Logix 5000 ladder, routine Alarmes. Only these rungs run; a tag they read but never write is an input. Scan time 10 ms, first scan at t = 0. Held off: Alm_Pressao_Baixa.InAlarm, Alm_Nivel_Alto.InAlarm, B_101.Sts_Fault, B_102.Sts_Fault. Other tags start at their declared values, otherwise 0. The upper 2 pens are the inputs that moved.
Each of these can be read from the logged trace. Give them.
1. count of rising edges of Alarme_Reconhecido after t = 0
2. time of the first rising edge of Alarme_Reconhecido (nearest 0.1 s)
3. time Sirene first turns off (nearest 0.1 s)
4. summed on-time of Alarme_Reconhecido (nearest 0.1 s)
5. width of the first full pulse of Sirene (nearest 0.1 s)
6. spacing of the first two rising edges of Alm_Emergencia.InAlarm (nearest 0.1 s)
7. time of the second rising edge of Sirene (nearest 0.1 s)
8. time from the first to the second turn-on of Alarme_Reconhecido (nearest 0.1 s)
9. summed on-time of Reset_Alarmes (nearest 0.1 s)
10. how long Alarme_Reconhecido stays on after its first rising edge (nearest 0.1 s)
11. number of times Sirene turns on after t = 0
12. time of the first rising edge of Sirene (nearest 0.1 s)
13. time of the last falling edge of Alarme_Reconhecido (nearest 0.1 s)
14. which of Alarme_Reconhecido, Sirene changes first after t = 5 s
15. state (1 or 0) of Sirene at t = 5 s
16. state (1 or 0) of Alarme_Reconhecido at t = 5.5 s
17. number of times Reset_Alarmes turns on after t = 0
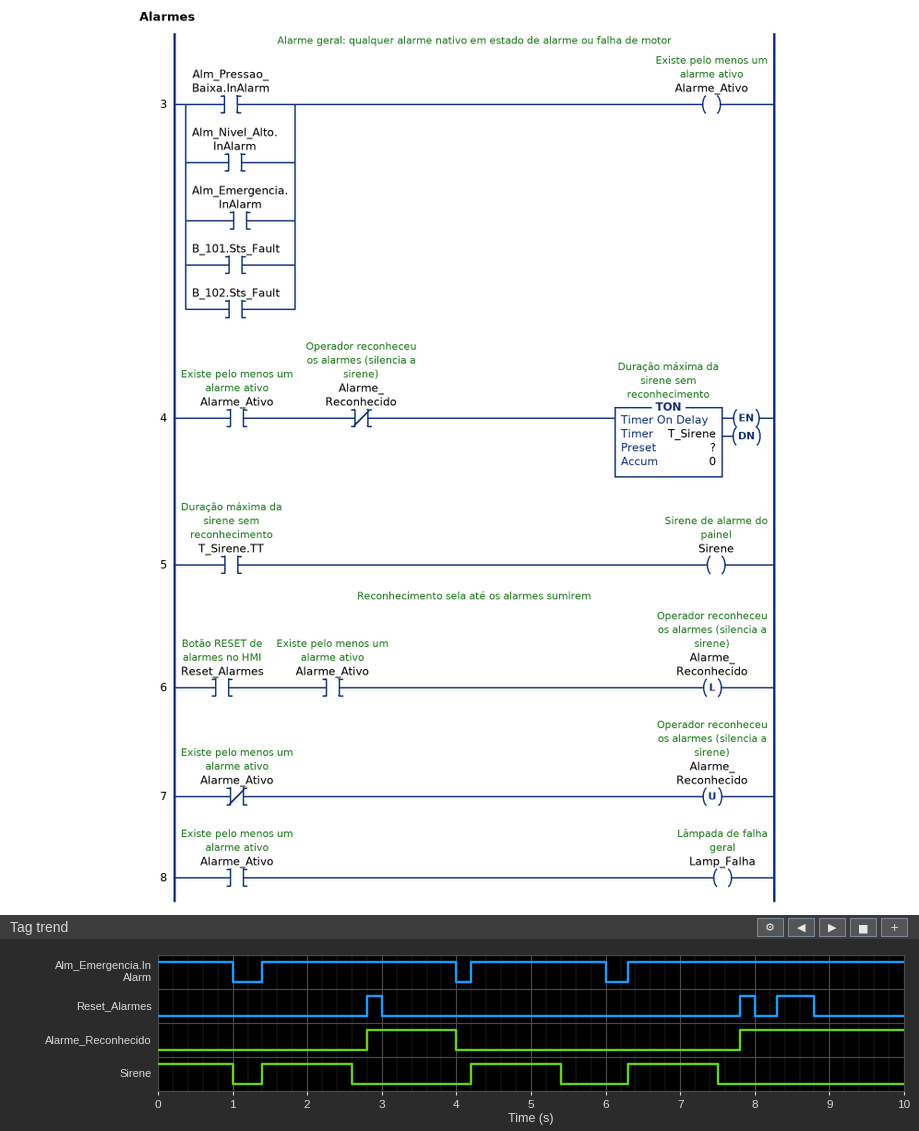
2
2.8 s
1.0 s
3.4 s
1.2 s
2.8 s
4.2 s
5.0 s
0.9 s
1.2 s
3
1.4 s
4.0 s
Sirene
1
0
3
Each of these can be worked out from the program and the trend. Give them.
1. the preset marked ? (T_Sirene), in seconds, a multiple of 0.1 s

1.2 s
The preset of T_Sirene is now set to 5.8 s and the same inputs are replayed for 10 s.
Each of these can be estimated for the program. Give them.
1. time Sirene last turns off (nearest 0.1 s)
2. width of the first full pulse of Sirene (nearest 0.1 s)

7.8 s
1.4 s
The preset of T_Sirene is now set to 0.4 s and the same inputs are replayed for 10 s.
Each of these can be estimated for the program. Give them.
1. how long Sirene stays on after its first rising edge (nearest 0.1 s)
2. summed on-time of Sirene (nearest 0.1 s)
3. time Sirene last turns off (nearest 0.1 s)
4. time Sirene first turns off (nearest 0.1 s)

0.4 s
1.6 s
6.7 s
0.4 s
